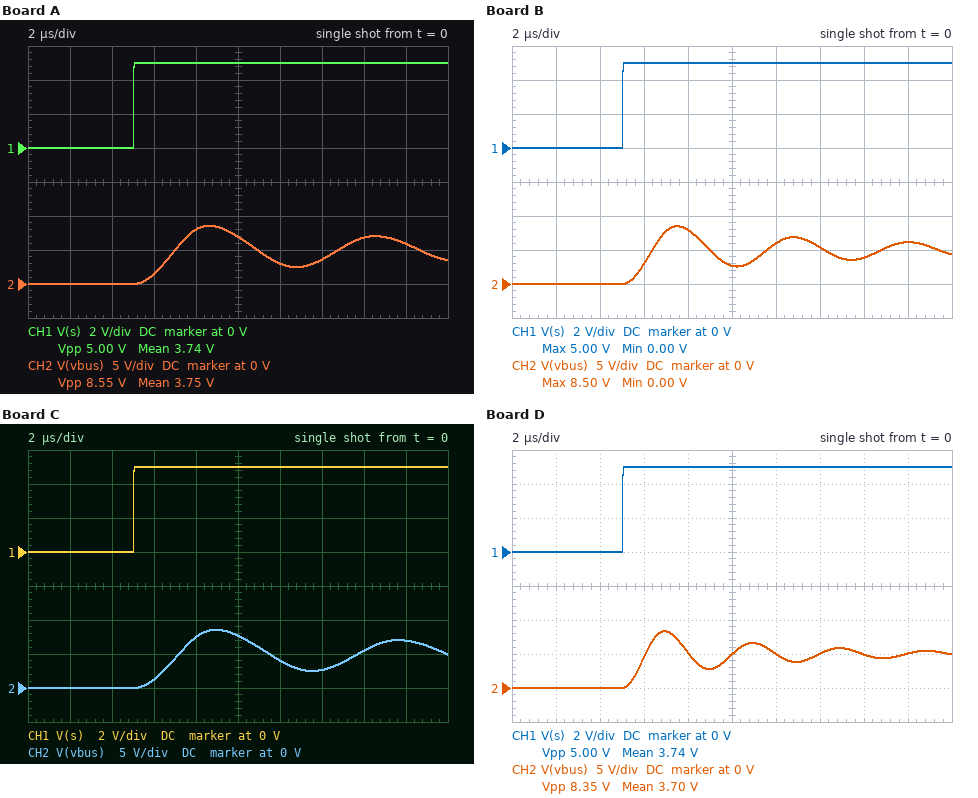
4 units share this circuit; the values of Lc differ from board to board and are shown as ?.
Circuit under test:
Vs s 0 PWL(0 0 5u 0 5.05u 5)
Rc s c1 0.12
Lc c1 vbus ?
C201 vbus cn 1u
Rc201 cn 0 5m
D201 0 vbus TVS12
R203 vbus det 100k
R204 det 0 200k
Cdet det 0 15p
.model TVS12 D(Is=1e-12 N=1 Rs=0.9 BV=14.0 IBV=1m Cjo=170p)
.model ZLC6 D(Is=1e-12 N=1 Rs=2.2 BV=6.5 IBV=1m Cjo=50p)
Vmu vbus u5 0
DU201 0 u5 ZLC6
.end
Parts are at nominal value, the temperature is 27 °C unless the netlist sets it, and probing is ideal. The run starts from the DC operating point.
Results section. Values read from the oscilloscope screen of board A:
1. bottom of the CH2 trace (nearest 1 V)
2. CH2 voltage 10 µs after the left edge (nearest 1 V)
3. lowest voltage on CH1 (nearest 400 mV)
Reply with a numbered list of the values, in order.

1. 0 V
2. 7 V
3. 0 V
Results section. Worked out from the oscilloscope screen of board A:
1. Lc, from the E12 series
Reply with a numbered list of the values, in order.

1. 1.5 µH
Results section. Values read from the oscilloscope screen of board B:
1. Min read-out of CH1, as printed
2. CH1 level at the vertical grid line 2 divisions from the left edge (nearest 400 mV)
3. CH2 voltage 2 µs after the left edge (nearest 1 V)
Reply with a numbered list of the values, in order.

1. 0.00 V
2. 0 V
3. 0 V
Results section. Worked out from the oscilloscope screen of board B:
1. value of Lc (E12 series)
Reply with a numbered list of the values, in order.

1. 680 nH
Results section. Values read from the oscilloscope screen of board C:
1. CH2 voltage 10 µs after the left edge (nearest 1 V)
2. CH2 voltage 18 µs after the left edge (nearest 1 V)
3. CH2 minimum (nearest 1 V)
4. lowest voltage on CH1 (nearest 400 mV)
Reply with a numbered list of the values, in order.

1. 8 V
2. 7 V
3. 0 V
4. 0 V
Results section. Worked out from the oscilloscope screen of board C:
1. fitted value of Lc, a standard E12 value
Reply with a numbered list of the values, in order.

1. 1.8 µH
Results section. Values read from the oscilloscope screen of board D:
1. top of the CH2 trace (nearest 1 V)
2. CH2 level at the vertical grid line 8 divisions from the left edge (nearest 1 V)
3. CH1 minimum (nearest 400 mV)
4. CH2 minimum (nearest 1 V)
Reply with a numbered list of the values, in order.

1. 8 V
2. 5 V
3. 0 V
4. 0 V
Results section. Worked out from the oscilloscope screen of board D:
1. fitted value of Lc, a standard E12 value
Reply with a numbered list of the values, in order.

1. 390 nH
